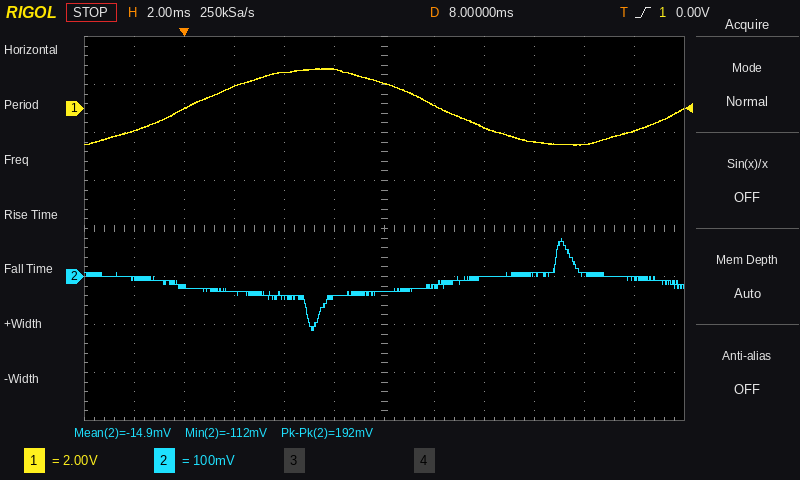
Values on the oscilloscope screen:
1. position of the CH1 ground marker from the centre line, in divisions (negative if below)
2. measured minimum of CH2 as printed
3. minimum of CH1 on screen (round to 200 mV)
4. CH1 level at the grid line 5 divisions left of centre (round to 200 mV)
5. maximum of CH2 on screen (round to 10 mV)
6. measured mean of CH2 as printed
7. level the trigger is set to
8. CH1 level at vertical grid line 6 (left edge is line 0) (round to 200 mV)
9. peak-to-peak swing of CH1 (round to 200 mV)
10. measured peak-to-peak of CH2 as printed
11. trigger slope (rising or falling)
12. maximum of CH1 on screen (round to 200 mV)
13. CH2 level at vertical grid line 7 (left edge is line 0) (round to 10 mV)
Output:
+2.5 div
-112 mV
-1.6 V
-1.0 V
80 mV
-14.9 mV
0.00 V
1.0 V
3.2 V
192 mV
rising
1.6 V
-20 mV
